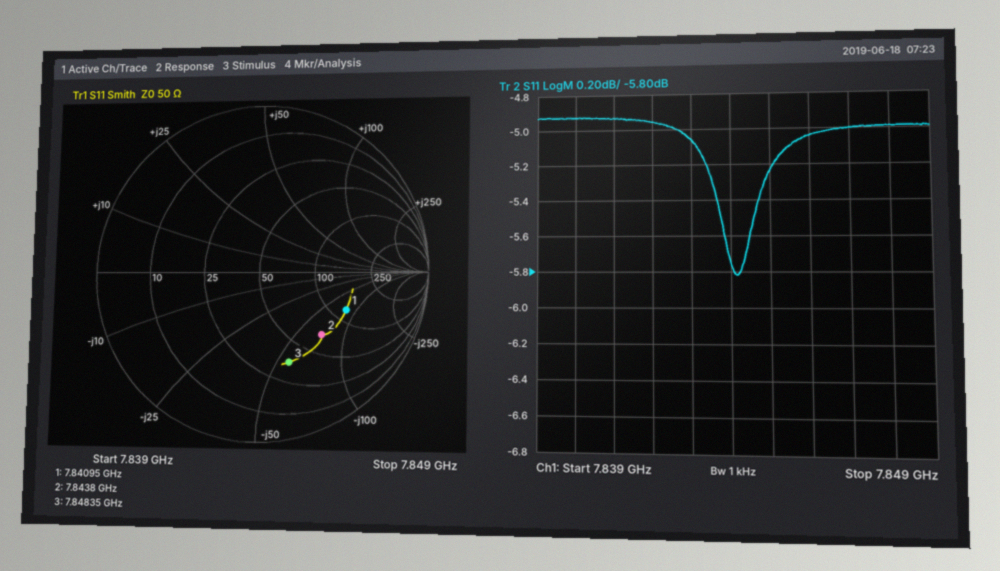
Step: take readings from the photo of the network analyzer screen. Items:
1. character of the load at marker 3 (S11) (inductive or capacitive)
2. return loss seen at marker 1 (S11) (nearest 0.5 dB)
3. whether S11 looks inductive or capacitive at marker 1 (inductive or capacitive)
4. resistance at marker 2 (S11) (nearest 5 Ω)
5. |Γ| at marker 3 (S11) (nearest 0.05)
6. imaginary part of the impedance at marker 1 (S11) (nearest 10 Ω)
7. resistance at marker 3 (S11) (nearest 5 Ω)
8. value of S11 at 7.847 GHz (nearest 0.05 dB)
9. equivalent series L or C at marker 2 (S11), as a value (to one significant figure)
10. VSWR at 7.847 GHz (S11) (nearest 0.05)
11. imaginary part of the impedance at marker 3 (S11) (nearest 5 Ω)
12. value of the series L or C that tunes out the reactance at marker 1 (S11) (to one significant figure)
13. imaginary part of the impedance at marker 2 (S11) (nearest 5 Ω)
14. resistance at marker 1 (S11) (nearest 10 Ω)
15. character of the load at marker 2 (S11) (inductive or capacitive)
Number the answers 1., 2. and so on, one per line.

1. capacitive
2. 5.0 dB
3. capacitive
4. 70 Ω
5. 0.55
6. -80 Ω
7. 35 Ω
8. -5.00 dB
9. 300 fF
10. 3.55
11. -55 Ω
12. 2 nH
13. -70 Ω
14. 120 Ω
15. capacitive
